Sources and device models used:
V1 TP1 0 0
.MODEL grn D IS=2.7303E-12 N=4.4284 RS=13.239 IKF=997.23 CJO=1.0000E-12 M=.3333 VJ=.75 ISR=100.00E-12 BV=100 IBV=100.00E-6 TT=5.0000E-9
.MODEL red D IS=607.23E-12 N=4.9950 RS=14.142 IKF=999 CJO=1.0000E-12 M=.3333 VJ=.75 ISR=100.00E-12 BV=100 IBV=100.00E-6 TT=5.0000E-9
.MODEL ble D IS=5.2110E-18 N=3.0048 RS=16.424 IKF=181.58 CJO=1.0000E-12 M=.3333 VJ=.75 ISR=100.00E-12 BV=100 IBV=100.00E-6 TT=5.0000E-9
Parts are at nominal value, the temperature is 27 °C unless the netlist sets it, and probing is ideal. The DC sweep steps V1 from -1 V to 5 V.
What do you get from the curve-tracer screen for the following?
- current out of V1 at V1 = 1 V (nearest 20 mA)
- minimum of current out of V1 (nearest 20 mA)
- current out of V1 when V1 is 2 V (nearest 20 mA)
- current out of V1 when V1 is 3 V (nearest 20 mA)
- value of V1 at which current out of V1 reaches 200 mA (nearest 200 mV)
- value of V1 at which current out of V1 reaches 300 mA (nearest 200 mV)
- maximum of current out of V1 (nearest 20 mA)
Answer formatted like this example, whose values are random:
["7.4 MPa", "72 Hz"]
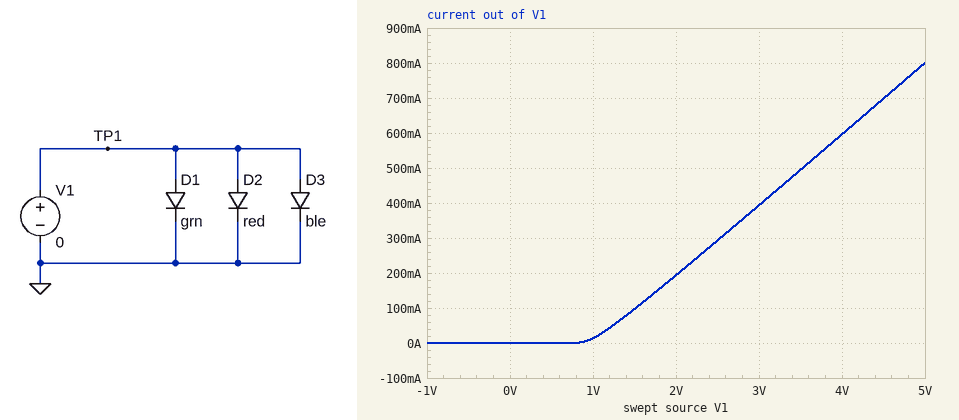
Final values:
["20 mA", "0 A", "200 mA", "400 mA", "2.0 V", "2.6 V", "800 mA"]
